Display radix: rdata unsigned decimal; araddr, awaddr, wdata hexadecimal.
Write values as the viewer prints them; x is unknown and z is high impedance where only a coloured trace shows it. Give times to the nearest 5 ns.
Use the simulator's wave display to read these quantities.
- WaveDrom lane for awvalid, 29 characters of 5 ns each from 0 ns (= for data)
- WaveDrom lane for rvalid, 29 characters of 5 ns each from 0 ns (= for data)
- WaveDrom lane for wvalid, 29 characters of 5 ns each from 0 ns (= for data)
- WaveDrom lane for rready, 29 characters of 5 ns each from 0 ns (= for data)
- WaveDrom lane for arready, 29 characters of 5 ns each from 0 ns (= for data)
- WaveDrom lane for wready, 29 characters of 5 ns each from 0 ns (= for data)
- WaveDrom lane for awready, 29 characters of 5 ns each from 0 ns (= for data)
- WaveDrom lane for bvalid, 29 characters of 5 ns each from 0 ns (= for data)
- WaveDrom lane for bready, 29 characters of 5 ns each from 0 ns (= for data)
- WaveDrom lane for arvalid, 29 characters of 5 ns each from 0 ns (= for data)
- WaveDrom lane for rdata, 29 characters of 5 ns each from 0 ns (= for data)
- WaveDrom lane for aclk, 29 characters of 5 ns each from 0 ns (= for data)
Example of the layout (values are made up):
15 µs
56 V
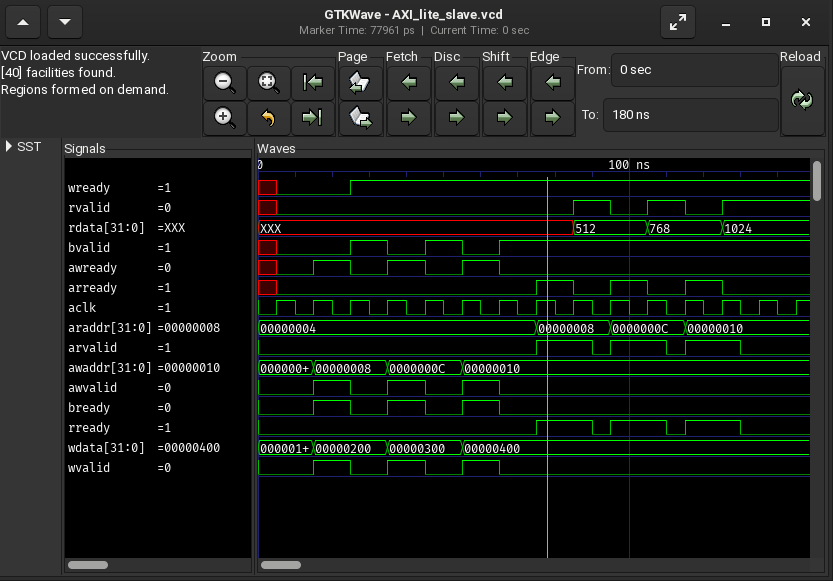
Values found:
{name: 'awvalid', wave: '0..1.0.1.0.1.0...............'}
{name: 'rvalid', wave: 'x0...............1.0.1.0.1...'}
{name: 'wvalid', wave: '0..1.0.1.0.1.0...............'}
{name: 'rready', wave: '0..............1..01..01..0..'}
{name: 'arready', wave: 'x0.............1.0.1.0.1.0...'}
{name: 'wready', wave: 'x0...1.......................'}
{name: 'awready', wave: 'x0.1.0.1.0.1.0...............'}
{name: 'bvalid', wave: 'x0...1.0.1.0.1...............'}
{name: 'bready', wave: '0..1.0.1.0.1.0...............'}
{name: 'arvalid', wave: '0..............1..01..01..0..'}
{name: 'rdata', wave: 'x................=...=...=...', data: '512 768 1024'}
{name: 'aclk', wave: '01010101010101010101010101010'}
